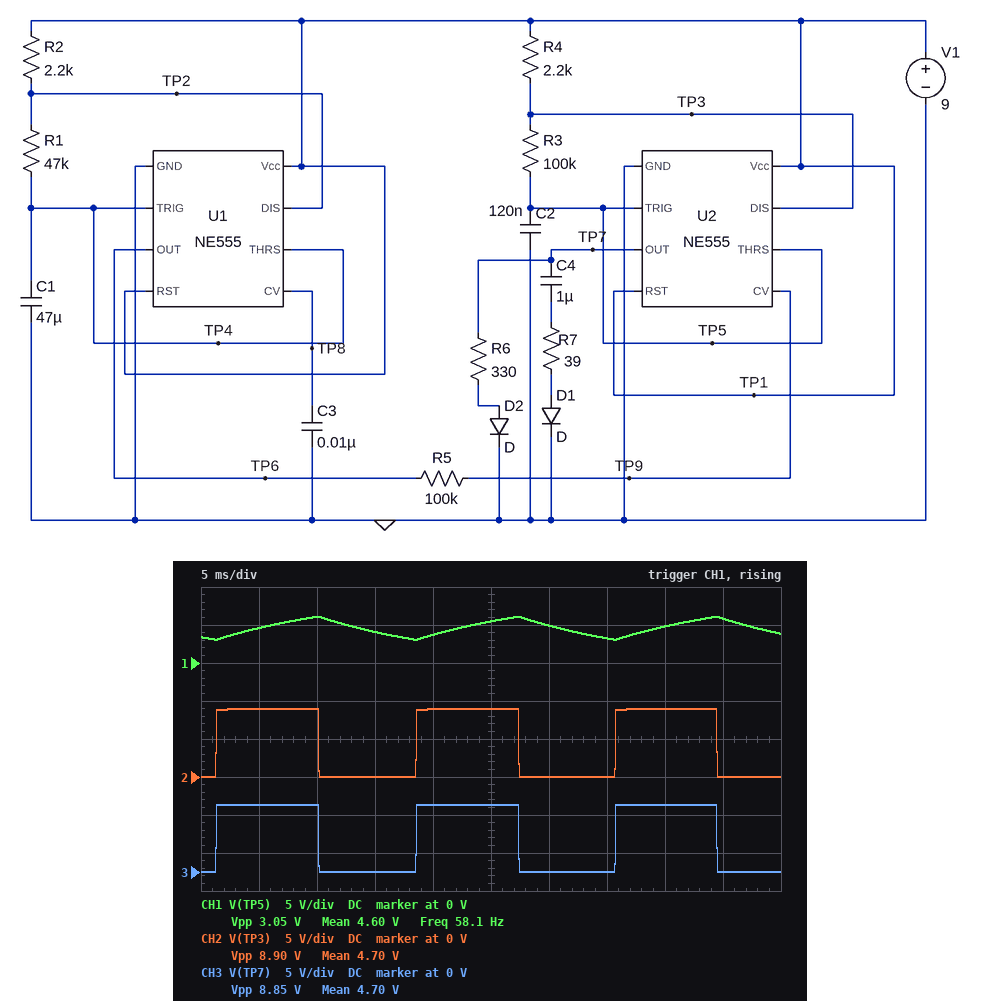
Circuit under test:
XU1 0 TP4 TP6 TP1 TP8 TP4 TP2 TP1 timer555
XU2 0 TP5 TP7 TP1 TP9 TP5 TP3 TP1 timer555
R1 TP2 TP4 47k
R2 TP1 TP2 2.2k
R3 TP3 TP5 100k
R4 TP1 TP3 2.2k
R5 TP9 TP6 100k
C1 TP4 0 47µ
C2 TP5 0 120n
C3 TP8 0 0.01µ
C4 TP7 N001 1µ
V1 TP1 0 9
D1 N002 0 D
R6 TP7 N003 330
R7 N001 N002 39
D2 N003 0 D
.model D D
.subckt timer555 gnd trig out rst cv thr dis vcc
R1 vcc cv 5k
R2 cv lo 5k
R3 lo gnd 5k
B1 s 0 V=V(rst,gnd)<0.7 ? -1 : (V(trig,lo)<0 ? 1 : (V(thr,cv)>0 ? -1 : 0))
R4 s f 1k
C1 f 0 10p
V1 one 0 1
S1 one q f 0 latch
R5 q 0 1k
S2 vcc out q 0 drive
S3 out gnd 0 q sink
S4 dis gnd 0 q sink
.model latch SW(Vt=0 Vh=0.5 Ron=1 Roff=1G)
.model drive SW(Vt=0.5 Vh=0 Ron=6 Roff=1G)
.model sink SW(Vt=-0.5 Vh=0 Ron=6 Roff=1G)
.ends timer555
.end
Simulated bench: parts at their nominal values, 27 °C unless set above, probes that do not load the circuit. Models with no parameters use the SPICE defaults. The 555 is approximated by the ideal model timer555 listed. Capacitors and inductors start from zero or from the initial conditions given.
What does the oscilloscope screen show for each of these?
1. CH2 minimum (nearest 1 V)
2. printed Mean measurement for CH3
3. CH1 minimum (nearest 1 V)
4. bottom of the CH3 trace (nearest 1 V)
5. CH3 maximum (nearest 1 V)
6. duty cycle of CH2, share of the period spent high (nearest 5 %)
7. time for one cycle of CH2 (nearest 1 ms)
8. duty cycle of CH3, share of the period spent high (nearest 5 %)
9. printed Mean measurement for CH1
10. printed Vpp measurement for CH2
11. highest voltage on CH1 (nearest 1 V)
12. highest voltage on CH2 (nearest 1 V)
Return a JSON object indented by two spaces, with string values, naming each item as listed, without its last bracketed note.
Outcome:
{
  "CH2 minimum": "0 V",
  "printed Mean measurement for CH3": "4.70 V",
  "CH1 minimum": "3 V",
  "bottom of the CH3 trace": "0 V",
  "CH3 maximum": "9 V",
  "duty cycle of CH2, share of the period spent high": "50 %",
  "time for one cycle of CH2": "17 ms",
  "duty cycle of CH3, share of the period spent high": "50 %",
  "printed Mean measurement for CH1": "4.60 V",
  "printed Vpp measurement for CH2": "8.90 V",
  "highest voltage on CH1": "6 V",
  "highest voltage on CH2": "9 V"
}
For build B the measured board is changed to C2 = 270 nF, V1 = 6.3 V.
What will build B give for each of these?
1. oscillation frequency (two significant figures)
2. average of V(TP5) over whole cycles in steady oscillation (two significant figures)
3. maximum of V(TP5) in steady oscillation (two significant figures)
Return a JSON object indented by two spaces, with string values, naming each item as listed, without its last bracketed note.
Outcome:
{
  "oscillation frequency": "26 Hz",
  "average of V(TP5) over whole cycles in steady oscillation": "3.2 V",
  "maximum of V(TP5) in steady oscillation": "4.3 V"
}
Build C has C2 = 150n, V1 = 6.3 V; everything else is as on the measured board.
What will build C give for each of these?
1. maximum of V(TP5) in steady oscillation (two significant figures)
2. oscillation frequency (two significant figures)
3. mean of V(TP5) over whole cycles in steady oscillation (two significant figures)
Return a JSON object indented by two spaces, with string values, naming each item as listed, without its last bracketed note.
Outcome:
{
  "maximum of V(TP5) in steady oscillation": "4.3 V",
  "oscillation frequency": "47 Hz",
  "mean of V(TP5) over whole cycles in steady oscillation": "3.2 V"
}
